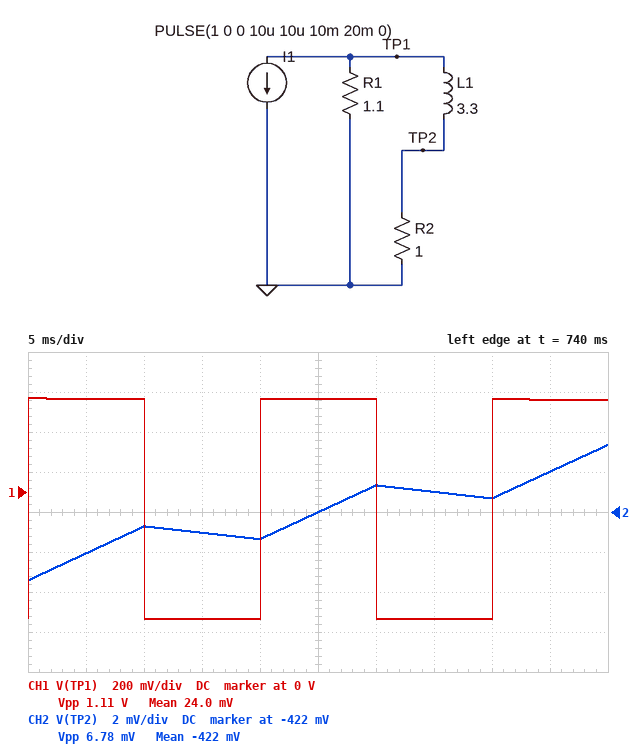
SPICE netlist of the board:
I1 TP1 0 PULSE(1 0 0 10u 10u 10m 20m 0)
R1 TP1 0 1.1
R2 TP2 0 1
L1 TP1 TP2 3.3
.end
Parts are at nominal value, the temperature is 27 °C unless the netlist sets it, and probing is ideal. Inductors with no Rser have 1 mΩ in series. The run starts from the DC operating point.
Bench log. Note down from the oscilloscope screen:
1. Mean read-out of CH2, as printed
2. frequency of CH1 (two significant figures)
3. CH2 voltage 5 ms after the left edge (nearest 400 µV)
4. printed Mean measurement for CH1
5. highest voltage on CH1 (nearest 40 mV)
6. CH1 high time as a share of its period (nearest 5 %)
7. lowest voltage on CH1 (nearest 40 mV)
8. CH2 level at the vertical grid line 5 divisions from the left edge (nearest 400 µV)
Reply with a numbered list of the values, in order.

1. -422 mV
2. 50 Hz
3. -424.0 mV
4. 24.0 mV
5. 480 mV
6. 50 %
7. -640 mV
8. -422.0 mV
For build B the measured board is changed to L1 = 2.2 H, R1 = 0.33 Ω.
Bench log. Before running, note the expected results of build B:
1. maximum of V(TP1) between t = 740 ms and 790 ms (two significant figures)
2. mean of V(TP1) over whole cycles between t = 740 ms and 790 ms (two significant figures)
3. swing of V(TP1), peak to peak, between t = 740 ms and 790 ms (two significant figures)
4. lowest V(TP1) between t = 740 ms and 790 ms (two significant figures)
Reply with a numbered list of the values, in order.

1. 67 mV
2. -98 mV
3. 330 mV
4. -260 mV
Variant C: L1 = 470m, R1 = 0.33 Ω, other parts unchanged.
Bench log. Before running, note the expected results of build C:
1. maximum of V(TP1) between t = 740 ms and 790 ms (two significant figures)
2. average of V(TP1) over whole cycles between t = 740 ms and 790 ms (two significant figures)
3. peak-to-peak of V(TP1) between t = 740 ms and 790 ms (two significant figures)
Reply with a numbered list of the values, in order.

1. 46 mV
2. -120 mV
3. 330 mV
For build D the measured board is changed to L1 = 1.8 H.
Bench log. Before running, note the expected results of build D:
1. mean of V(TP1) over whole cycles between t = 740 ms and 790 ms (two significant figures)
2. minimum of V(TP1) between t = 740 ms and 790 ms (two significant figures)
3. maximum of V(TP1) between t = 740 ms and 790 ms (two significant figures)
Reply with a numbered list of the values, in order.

1. -140 mV
2. -700 mV
3. 410 mV
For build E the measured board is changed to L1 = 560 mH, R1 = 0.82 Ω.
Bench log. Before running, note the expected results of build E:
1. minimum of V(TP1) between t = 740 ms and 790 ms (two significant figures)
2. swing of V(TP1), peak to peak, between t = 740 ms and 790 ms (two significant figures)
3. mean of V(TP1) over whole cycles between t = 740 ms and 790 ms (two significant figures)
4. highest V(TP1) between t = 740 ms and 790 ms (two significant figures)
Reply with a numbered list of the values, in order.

1. -620 mV
2. 830 mV
3. -210 mV
4. 200 mV
